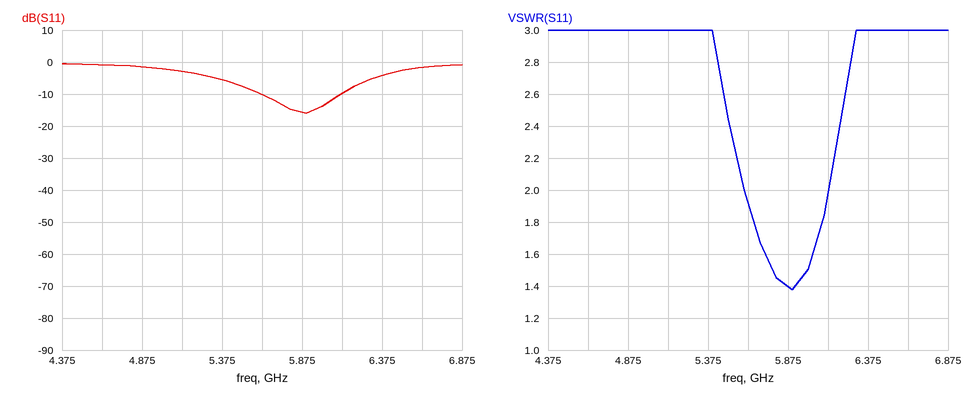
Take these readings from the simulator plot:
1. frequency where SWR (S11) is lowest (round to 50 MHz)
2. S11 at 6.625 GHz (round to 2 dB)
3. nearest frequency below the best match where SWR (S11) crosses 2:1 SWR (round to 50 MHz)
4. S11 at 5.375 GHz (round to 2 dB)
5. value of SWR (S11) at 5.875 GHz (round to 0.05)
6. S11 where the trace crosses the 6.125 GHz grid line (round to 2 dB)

5.90 GHz
-2 dB
5.60 GHz
-6 dB
1.40
-10 dB
